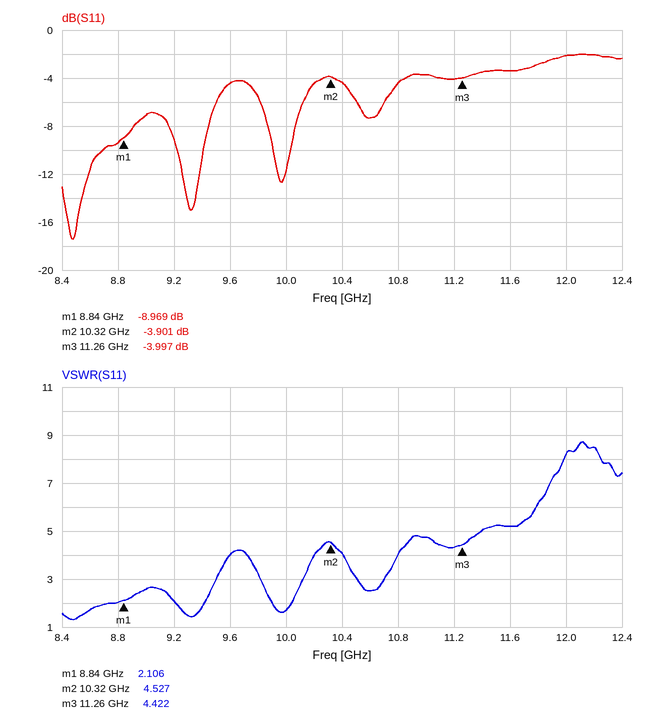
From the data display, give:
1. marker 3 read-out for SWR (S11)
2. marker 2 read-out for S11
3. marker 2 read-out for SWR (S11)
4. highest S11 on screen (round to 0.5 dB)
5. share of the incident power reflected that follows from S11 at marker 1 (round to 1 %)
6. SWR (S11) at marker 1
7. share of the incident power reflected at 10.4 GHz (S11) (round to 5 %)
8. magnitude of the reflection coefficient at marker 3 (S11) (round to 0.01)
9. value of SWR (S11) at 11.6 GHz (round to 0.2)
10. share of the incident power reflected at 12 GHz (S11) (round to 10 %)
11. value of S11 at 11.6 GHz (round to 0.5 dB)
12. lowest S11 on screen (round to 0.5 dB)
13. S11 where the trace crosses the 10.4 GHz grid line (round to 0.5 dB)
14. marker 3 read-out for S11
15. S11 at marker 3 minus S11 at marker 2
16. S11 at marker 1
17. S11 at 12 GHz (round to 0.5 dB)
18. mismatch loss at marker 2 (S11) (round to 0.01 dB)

4.422
-3.901 dB
4.527
-2.0 dB
13 %
2.106
35 %
0.63
5.2
60 %
-3.5 dB
-17.5 dB
-4.5 dB
-3.997 dB
-0.096 dB
-8.969 dB
-2.0 dB
2.27 dB
